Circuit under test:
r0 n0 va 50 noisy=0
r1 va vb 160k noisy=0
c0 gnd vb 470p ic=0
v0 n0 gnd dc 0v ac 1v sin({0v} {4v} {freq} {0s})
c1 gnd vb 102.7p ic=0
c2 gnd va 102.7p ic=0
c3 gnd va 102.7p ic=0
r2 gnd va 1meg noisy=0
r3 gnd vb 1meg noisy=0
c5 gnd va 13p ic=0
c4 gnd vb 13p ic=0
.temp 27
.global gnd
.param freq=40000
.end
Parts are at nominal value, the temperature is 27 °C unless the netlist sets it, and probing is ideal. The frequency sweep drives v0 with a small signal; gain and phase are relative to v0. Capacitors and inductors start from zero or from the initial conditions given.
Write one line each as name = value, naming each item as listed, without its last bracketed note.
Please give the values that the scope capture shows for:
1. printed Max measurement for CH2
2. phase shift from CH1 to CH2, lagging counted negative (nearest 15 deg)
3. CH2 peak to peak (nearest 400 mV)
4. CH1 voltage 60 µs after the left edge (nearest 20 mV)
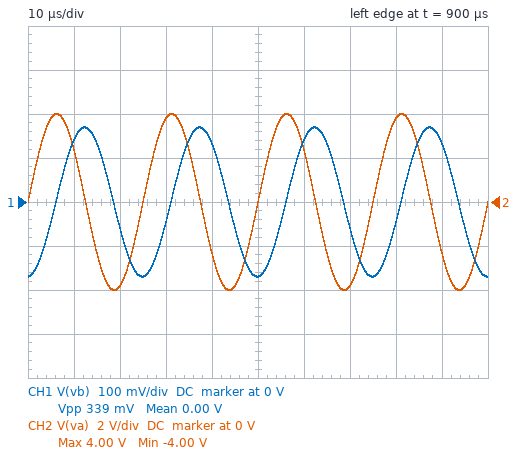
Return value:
printed Max measurement for CH2 = 4.00 V
phase shift from CH1 to CH2, lagging counted negative = 90 deg
CH2 peak to peak = 8.0 V
CH1 voltage 60 µs after the left edge = 140 mV
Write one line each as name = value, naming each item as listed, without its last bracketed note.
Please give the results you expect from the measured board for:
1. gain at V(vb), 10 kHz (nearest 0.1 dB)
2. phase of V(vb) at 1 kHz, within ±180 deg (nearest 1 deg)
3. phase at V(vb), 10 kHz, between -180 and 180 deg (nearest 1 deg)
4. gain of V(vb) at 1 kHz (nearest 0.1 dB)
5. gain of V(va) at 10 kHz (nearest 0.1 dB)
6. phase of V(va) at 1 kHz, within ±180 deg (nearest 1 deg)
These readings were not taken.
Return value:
gain at V(vb), 10 kHz = -15.6 dB
phase of V(vb) at 1 kHz, within ±180 deg = -27 deg
phase at V(vb), 10 kHz, between -180 and 180 deg = -79 deg
gain of V(vb) at 1 kHz = -2.3 dB
gain of V(va) at 10 kHz = 0 dB
phase of V(va) at 1 kHz, within ±180 deg = 0 deg
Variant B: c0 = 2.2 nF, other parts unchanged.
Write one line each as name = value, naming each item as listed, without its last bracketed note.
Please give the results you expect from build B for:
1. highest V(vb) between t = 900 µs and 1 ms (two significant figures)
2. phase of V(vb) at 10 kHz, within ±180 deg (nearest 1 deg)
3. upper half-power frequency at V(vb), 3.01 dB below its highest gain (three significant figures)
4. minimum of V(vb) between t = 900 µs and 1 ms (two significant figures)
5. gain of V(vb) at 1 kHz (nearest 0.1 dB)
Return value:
highest V(vb) between t = 900 µs and 1 ms = 45 mV
phase of V(vb) at 10 kHz, within ±180 deg = -87 deg
upper half-power frequency at V(vb), 3.01 dB below its highest gain = 498 Hz
minimum of V(vb) between t = 900 µs and 1 ms = -41 mV
gain of V(vb) at 1 kHz = -8.3 dB
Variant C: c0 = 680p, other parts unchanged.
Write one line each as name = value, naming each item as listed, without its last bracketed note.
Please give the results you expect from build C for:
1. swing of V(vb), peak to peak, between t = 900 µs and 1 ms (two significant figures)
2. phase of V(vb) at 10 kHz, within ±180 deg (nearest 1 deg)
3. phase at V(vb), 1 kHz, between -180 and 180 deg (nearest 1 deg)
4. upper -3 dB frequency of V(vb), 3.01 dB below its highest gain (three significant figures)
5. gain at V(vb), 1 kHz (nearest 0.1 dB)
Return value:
swing of V(vb), peak to peak, between t = 900 µs and 1 ms = 250 mV
phase of V(vb) at 10 kHz, within ±180 deg = -82 deg
phase at V(vb), 1 kHz, between -180 and 180 deg = -35 deg
upper -3 dB frequency of V(vb), 3.01 dB below its highest gain = 1.45 kHz
gain at V(vb), 1 kHz = -3.0 dB
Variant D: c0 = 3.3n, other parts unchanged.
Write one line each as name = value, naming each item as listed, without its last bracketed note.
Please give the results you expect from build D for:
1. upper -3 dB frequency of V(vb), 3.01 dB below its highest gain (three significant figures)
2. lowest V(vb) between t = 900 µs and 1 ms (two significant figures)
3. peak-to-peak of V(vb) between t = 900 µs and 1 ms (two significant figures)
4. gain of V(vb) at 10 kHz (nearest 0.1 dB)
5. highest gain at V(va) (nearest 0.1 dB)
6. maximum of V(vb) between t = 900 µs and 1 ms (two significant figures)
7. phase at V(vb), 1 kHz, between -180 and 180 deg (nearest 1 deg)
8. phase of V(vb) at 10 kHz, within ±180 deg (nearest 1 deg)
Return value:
upper -3 dB frequency of V(vb), 3.01 dB below its highest gain = 338 Hz
lowest V(vb) between t = 900 µs and 1 ms = -26 mV
peak-to-peak of V(vb) between t = 900 µs and 1 ms = 59 mV
gain of V(vb) at 10 kHz = -30.7 dB
highest gain at V(va) = 0 dB
maximum of V(vb) between t = 900 µs and 1 ms = 33 mV
phase at V(vb), 1 kHz, between -180 and 180 deg = -71 deg
phase of V(vb) at 10 kHz, within ±180 deg = -88 deg
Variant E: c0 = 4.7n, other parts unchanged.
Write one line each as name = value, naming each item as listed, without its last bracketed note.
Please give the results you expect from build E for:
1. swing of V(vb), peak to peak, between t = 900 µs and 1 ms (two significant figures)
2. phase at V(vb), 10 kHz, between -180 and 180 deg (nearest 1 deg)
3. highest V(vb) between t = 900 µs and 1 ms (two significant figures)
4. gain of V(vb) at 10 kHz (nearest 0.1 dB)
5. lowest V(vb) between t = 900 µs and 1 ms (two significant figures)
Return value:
swing of V(vb), peak to peak, between t = 900 µs and 1 ms = 42 mV
phase at V(vb), 10 kHz, between -180 and 180 deg = -89 deg
highest V(vb) between t = 900 µs and 1 ms = 26 mV
gain of V(vb) at 10 kHz = -33.7 dB
lowest V(vb) between t = 900 µs and 1 ms = -16 mV
